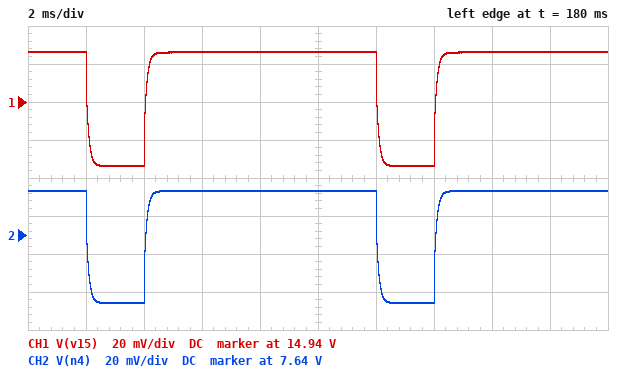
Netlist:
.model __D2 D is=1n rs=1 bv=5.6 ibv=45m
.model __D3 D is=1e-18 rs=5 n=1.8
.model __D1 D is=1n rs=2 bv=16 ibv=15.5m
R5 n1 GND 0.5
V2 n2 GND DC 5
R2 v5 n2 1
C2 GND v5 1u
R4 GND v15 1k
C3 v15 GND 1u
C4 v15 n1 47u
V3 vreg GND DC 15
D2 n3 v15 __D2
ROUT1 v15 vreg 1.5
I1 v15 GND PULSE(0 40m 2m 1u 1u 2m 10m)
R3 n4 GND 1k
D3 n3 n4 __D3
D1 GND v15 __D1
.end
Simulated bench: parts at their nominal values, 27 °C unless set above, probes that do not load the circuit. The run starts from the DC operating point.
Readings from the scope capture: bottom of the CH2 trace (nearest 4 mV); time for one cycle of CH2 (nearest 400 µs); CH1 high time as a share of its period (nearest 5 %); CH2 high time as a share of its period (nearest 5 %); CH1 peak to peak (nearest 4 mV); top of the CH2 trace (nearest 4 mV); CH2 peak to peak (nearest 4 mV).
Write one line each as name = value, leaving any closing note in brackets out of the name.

bottom of the CH2 trace = 7.604 V
time for one cycle of CH2 = 10.0 ms
CH1 high time as a share of its period = 80 %
CH2 high time as a share of its period = 80 %
CH1 peak to peak = 60 mV
top of the CH2 trace = 7.664 V
CH2 peak to peak = 60 mV
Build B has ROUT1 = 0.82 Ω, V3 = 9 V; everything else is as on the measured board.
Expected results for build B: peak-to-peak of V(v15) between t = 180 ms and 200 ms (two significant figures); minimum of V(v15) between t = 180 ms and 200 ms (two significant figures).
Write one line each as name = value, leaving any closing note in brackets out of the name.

peak-to-peak of V(v15) between t = 180 ms and 200 ms = 33 mV
minimum of V(v15) between t = 180 ms and 200 ms = 9.0 V
